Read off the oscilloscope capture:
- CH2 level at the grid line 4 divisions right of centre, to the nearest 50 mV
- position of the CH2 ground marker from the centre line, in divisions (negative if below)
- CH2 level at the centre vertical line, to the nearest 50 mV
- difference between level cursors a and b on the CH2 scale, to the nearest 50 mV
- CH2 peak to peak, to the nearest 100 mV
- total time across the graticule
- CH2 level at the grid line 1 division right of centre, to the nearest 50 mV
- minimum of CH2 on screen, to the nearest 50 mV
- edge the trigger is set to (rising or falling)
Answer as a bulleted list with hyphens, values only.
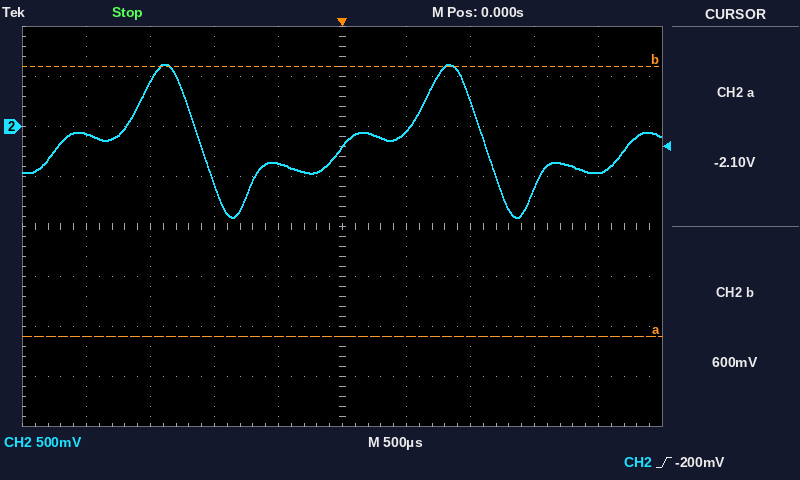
- -450 mV
- +2.0 div
- -200 mV
- 2.70 V
- 1.50 V
- 5 ms
- -50 mV
- -900 mV
- rising
